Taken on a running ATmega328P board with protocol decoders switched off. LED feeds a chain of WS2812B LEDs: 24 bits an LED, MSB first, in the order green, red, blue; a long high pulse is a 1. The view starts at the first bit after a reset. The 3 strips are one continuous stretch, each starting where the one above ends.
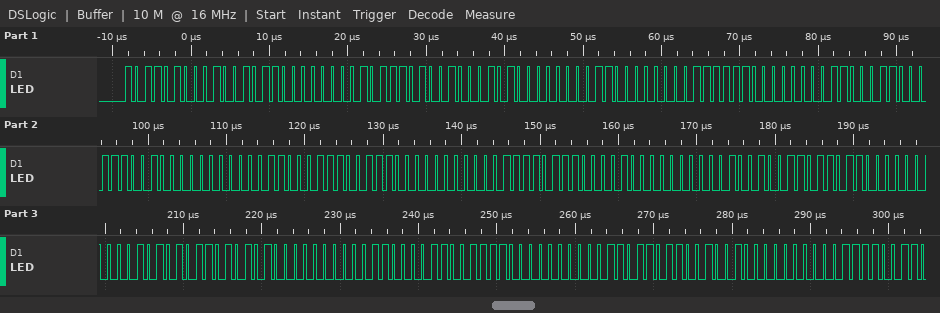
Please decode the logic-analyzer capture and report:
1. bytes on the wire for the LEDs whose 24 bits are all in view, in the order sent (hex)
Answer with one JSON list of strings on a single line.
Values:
["B4 4B 00 BA 45 00 C0 3F 00 C6 39 00 18 E7 00 1E E1 00 24 DB 00 2A D5 00 30 CF 00 36 C9 00"]
